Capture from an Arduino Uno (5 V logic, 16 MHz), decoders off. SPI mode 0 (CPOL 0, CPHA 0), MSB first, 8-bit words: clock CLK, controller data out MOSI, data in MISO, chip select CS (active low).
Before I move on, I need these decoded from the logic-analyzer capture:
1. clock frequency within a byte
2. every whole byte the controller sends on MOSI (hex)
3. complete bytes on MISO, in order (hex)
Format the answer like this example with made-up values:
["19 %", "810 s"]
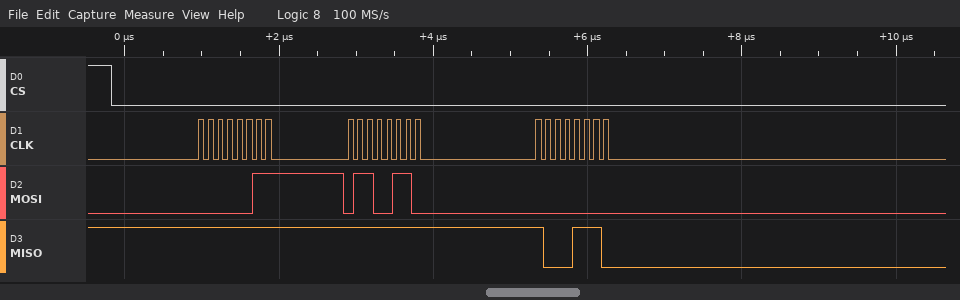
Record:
["8 MHz", "0x03 0x66 0x00", "0xFF 0xFF 0x8E"]
